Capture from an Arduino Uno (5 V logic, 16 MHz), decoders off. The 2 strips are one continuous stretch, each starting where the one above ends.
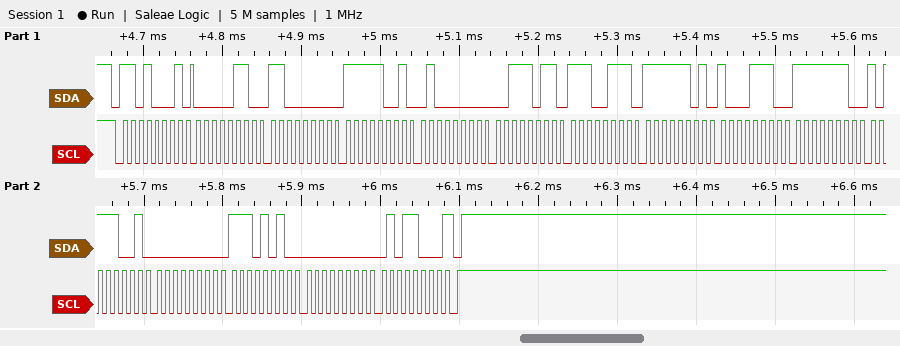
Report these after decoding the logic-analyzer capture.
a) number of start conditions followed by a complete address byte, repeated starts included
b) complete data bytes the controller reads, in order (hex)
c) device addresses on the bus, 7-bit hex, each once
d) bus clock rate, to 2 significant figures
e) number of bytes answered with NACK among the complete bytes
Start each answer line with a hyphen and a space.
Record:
- 1
- 06 C0 F9 40 3B E7 FD 8E FE B9 00 EA 00 58
- 0x68
- 100 kHz
- 1
